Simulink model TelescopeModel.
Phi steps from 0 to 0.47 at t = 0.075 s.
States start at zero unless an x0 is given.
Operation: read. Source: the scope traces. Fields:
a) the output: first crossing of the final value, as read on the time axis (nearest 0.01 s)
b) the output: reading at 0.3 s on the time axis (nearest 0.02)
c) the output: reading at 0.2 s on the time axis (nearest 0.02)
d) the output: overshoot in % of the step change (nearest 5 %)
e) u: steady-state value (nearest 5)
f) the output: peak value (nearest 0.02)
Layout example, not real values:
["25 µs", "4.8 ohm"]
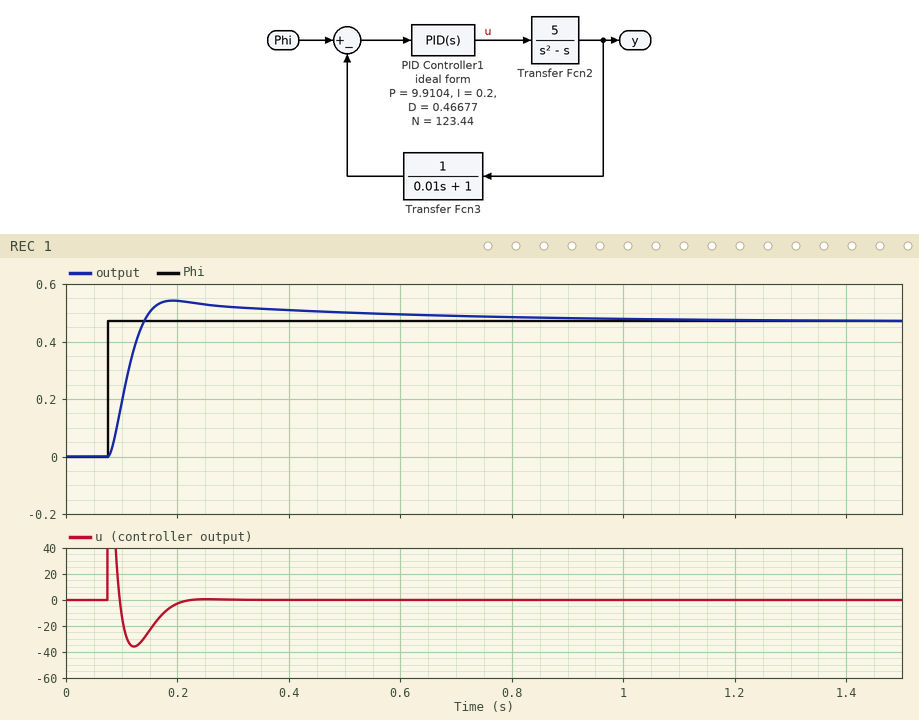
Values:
["0.14 s", "0.52", "0.54", "15 %", "0", "0.54"]
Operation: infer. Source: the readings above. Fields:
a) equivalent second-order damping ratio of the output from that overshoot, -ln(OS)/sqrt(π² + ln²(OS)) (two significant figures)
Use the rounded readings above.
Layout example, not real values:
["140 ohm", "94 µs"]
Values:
["0.52"]
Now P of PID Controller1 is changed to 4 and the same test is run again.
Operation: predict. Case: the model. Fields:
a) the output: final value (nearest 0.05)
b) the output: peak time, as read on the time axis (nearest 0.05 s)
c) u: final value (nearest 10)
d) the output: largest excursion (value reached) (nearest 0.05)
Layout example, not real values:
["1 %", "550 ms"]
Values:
["0.45", "0.45 s", "0", "0.60"]
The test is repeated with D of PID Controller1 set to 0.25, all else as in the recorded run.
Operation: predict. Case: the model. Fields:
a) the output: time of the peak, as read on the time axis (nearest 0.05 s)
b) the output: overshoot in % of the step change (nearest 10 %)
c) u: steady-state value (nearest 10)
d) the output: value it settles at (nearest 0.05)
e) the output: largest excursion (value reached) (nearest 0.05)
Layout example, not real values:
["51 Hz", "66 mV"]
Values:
["0.30 s", "30 %", "0", "0.45", "0.60"]
